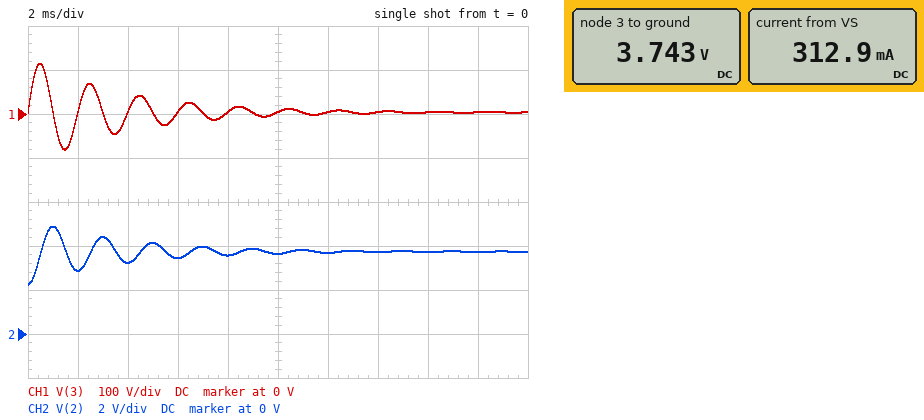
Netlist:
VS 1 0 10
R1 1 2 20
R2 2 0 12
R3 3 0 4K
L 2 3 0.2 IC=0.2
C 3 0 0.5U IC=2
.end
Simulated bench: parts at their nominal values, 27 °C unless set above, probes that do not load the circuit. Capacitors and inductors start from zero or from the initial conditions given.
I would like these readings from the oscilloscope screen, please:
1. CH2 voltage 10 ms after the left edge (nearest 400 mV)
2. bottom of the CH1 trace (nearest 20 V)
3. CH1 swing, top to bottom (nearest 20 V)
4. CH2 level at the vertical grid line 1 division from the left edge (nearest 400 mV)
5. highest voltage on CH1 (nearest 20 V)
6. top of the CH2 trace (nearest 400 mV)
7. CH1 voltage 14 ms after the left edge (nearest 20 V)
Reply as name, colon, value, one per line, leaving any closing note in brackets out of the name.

CH2 voltage 10 ms after the left edge: 3.6 V
bottom of the CH1 trace: -80 V
CH1 swing, top to bottom: 200 V
CH2 level at the vertical grid line 1 division from the left edge: 2.8 V
highest voltage on CH1: 120 V
top of the CH2 trace: 4.8 V
CH1 voltage 14 ms after the left edge: 0 V
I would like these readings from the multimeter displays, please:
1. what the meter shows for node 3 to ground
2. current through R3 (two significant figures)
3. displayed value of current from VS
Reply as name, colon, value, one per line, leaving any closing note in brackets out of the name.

what the meter shows for node 3 to ground: 3.743 V
current through R3: 940 µA
displayed value of current from VS: 312.9 mA
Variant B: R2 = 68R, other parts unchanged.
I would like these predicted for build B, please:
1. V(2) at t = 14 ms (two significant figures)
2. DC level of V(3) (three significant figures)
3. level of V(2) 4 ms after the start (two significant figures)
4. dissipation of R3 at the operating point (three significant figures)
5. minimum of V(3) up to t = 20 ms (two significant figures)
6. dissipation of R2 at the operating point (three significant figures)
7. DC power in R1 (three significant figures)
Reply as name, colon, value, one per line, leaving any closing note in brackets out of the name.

V(2) at t = 14 ms: 7.6 V
DC level of V(3): 7.70 V
level of V(2) 4 ms after the start: 6.7 V
dissipation of R3 at the operating point: 14.8 mW
minimum of V(3) up to t = 20 ms: -74 V
dissipation of R2 at the operating point: 871 mW
DC power in R1: 265 mW
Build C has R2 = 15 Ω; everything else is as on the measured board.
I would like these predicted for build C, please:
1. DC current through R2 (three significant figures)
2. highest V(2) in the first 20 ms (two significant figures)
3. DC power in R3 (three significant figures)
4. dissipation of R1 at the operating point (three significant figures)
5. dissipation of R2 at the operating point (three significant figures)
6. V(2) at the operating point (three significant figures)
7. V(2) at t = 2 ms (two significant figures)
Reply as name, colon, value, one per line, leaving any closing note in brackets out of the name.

DC current through R2: 285 mA
highest V(2) in the first 20 ms: 5.6 V
DC power in R3: 4.57 mW
dissipation of R1 at the operating point: 1.64 W
dissipation of R2 at the operating point: 1.22 W
V(2) at the operating point: 4.28 V
V(2) at t = 2 ms: 3.3 V
